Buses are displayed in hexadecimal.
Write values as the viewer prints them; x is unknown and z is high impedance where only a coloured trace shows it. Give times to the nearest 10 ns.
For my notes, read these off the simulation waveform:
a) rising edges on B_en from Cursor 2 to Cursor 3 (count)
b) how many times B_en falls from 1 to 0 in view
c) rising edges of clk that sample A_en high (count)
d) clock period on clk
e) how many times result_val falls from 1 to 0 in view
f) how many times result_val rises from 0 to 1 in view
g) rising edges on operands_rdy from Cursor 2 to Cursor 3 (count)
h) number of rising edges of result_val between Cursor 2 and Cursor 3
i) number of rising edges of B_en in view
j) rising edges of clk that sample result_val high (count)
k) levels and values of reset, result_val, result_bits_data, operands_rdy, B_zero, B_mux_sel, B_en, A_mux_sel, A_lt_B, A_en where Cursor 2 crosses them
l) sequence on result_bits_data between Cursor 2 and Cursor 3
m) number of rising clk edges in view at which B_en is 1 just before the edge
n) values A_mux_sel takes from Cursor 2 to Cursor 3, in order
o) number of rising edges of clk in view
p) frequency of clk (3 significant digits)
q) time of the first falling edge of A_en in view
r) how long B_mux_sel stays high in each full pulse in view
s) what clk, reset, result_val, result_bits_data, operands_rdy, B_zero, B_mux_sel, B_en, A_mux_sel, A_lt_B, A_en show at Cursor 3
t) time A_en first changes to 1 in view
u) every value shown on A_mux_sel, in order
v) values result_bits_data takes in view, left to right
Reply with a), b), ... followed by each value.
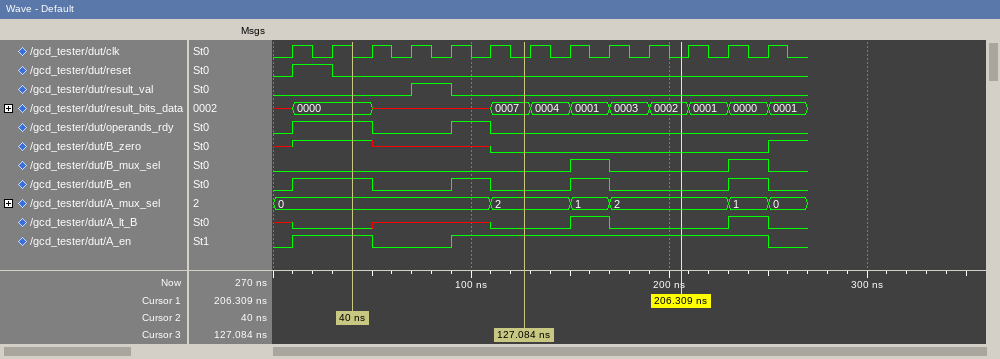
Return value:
a) 1
b) 4
c) 10
d) 20 ns
e) 1
f) 1
g) 1
h) 1
i) 4
j) 1
k) reset=0, result_val=0, result_bits_data=0000, operands_rdy=1, B_zero=1, B_mux_sel=0, B_en=1, A_mux_sel=0, A_lt_B=0, A_en=1
l) 0000, x, 0007
m) 5
n) 0, 2
o) 13
p) 50.0 MHz
q) 50 ns
r) 20 ns, 20 ns
s) clk=0, reset=0, result_val=0, result_bits_data=0007, operands_rdy=0, B_zero=0, B_mux_sel=0, B_en=0, A_mux_sel=2, A_lt_B=0, A_en=1
t) 10 ns
u) 0, 2, 1, 2, 1, 0
v) x, 0000, x, 0007, 0004, 0001, 0003, 0002, 0001, 0000, 0001
